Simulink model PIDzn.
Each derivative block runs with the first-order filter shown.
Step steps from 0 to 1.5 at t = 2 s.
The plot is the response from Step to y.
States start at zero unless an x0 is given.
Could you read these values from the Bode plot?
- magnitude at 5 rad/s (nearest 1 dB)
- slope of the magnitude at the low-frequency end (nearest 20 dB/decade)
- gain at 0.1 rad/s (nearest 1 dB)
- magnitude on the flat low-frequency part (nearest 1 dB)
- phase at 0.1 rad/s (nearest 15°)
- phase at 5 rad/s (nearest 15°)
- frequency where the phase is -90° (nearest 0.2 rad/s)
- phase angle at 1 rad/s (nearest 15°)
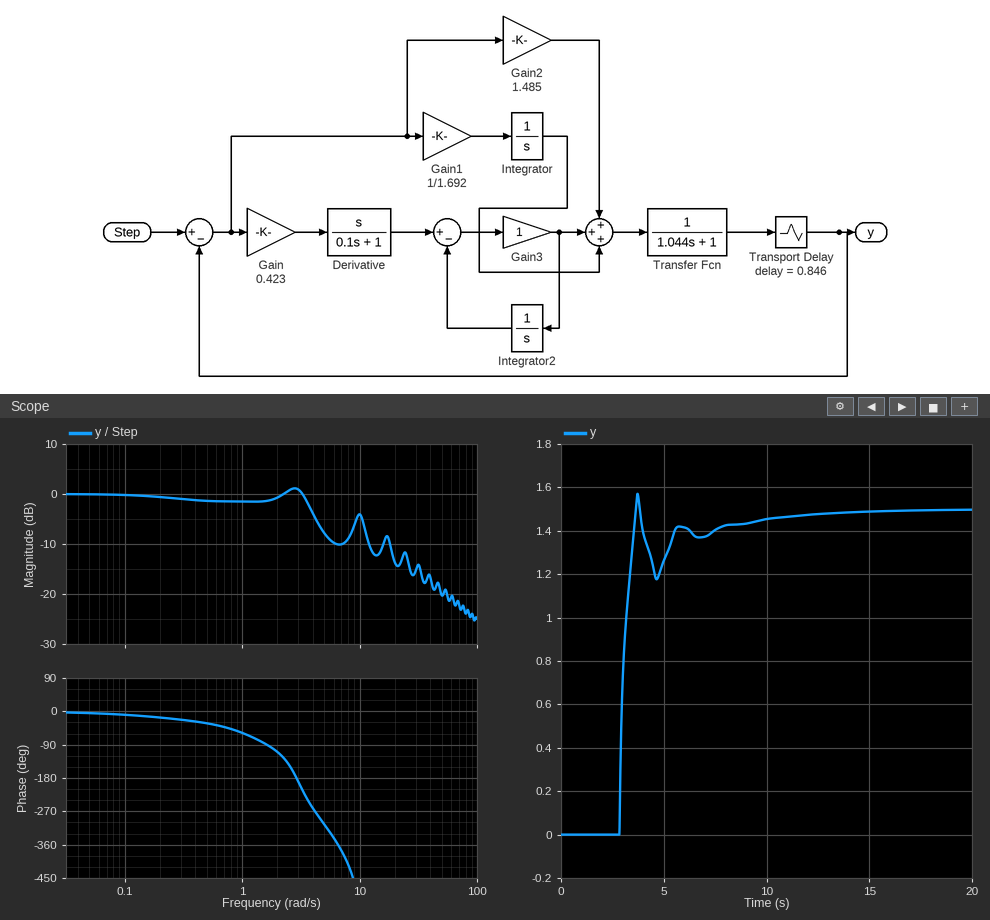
-8 dB
0 dB/decade
0 dB
0 dB
-15°
-300°
1.6 rad/s
-60°
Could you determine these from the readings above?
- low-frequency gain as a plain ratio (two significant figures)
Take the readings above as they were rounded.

1.0
